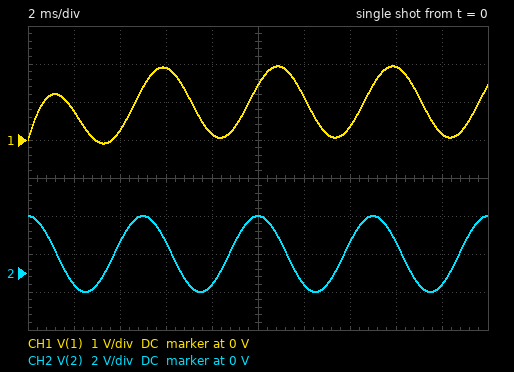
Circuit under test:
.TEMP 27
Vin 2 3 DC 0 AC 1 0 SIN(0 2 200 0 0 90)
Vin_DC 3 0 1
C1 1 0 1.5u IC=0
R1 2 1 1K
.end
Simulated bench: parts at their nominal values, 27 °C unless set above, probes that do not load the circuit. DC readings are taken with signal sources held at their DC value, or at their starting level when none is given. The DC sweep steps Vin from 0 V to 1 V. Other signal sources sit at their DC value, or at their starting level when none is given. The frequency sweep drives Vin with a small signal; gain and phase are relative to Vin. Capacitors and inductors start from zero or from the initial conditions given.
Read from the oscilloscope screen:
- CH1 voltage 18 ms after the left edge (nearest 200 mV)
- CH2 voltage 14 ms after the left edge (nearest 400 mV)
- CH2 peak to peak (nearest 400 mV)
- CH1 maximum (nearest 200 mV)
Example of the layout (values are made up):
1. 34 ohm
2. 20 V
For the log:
1. 200 mV
2. 1.6 V
3. 4.0 V
4. 2.0 V
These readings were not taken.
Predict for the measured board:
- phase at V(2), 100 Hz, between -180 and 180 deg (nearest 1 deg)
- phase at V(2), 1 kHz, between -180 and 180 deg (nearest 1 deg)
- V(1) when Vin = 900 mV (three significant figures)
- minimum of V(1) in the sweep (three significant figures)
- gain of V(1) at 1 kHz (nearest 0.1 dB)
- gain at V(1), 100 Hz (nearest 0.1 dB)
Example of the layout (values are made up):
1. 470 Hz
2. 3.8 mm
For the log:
1. 0 deg
2. 0 deg
3. 1.90 V
4. 1.00 V
5. -19.5 dB
6. -2.8 dB
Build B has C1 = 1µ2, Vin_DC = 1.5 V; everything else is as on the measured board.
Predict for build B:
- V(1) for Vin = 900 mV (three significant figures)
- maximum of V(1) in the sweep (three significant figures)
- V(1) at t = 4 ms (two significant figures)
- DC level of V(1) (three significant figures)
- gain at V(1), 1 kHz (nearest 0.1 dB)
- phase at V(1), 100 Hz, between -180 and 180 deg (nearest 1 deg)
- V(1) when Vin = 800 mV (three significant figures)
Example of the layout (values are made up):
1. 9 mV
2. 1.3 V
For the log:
1. 2.40 V
2. 2.50 V
3. 740 mV
4. 1.50 V
5. -17.6 dB
6. -37 deg
7. 2.30 V
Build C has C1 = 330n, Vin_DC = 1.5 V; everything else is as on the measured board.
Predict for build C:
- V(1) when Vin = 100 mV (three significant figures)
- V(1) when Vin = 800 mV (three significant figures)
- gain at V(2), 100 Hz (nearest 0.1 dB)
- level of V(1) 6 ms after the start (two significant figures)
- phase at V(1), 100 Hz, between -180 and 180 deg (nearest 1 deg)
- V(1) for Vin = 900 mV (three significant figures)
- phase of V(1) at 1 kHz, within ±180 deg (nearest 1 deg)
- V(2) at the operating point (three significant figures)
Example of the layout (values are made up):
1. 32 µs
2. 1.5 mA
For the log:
1. 1.60 V
2. 2.30 V
3. 0 dB
4. 2.7 V
5. -12 deg
6. 2.40 V
7. -64 deg
8. 1.50 V
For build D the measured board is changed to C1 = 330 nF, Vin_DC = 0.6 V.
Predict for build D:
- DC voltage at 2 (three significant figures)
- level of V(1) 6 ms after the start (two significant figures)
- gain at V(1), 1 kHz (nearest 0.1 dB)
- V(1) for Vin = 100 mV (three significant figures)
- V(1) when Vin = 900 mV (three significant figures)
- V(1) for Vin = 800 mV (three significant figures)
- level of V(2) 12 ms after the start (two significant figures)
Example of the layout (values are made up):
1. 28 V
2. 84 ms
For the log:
1. 600 mV
2. 1.8 V
3. -7.2 dB
4. 700 mV
5. 1.50 V
6. 1.40 V
7. -1.0 V
